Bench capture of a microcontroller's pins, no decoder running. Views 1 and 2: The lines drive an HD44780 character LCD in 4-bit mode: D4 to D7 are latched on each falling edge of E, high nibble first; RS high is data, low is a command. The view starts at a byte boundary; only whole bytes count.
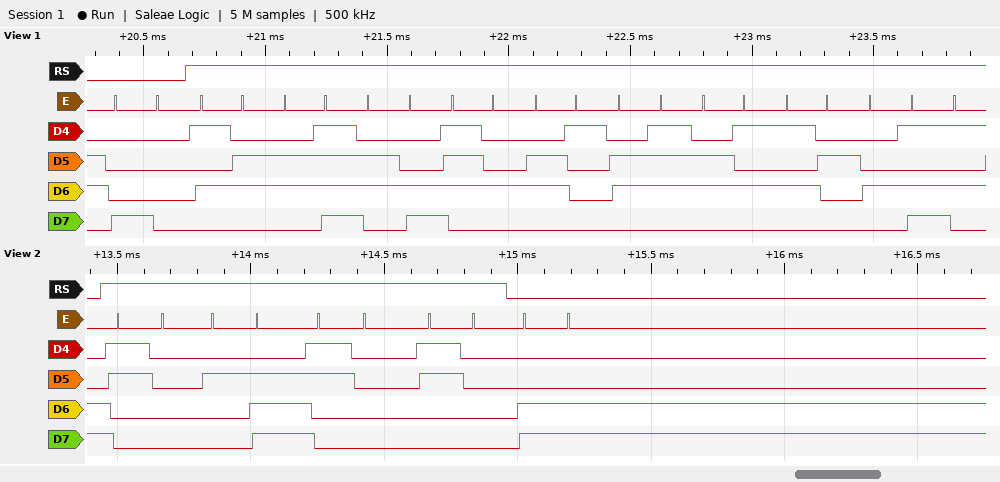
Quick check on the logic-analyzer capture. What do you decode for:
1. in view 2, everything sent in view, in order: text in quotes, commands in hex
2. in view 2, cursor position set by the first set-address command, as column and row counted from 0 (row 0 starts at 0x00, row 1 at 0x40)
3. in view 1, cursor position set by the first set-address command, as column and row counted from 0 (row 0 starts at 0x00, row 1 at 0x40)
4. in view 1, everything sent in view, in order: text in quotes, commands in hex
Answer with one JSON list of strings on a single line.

["\"0.00\" 0xCC", "column 12, row 1", "column 0, row 0", "0x80 \"VoltageRM\""]
